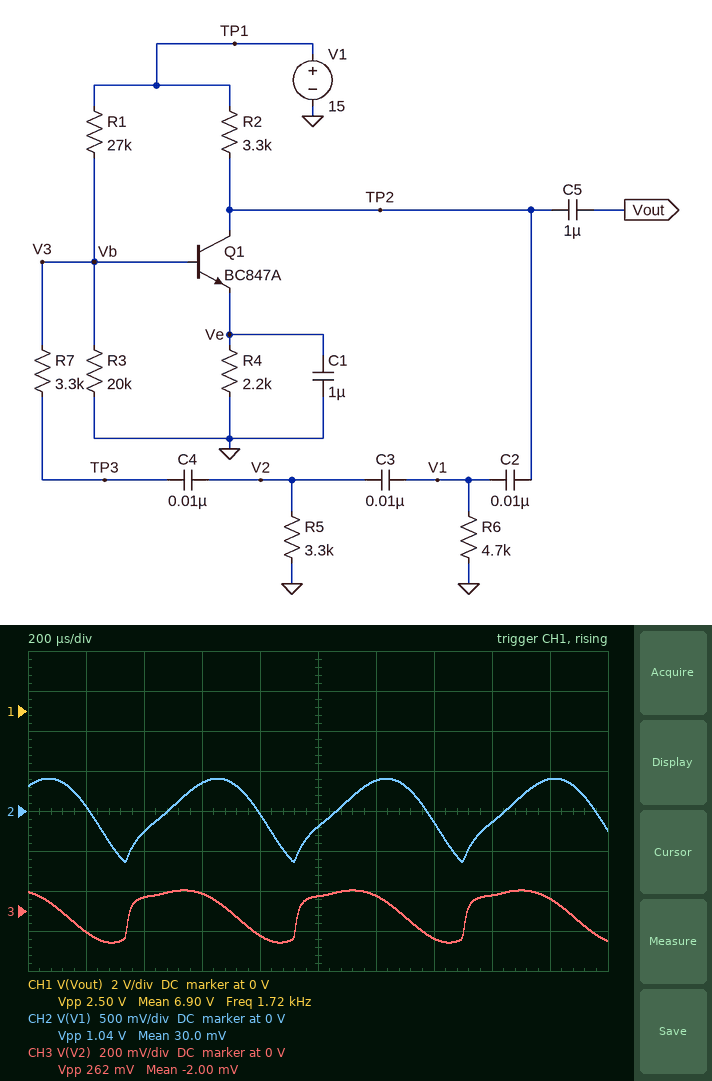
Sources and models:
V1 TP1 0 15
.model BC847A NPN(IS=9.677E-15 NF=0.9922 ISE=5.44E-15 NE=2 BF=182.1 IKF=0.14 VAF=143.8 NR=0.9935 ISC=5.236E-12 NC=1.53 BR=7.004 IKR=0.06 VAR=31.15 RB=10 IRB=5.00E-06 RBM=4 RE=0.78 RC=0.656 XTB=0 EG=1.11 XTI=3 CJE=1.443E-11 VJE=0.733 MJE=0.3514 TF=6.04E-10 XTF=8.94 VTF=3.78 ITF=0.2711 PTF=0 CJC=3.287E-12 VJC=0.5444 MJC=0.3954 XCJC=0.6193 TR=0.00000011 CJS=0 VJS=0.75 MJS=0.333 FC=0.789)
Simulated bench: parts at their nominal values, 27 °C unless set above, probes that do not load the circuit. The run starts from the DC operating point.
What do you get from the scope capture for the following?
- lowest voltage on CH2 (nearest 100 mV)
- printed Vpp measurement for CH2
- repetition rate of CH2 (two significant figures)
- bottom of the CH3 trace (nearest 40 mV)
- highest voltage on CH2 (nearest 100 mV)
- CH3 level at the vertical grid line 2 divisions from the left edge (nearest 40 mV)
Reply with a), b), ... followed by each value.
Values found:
a) -600 mV
b) 1.04 V
c) 1.7 kHz
d) -160 mV
e) 400 mV
f) 80 mV
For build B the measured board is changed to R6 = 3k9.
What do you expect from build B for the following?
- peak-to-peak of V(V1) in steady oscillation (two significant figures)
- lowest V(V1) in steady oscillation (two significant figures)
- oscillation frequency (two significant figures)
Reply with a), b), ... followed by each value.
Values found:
a) 970 mV
b) -600 mV
c) 1.8 kHz
